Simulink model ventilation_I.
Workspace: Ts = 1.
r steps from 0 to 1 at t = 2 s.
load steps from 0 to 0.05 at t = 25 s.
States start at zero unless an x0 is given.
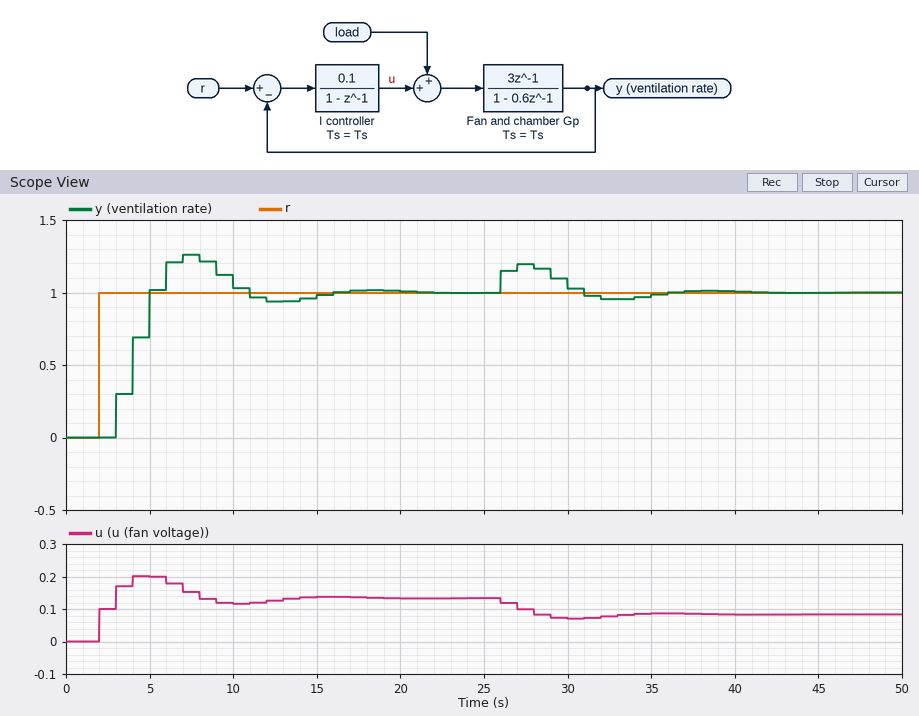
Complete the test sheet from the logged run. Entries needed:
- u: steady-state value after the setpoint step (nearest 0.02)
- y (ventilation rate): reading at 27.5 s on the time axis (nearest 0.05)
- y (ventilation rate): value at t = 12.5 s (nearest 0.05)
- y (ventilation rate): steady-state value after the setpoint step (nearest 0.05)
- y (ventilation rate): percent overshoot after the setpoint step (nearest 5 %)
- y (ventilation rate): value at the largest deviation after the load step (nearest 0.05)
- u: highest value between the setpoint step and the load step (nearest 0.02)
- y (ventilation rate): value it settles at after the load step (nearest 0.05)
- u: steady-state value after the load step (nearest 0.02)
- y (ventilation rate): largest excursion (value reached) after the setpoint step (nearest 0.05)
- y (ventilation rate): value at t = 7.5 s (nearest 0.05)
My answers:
0.14
1.20
0.95
1.00
25 %
1.20
0.20
1.00
0.08
1.25
1.25
